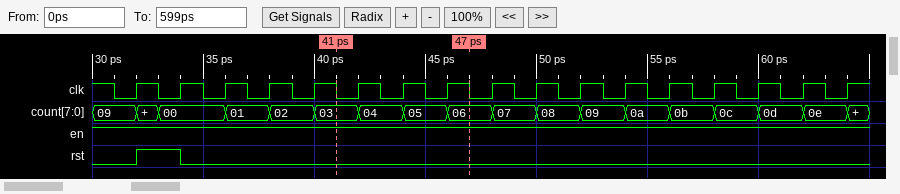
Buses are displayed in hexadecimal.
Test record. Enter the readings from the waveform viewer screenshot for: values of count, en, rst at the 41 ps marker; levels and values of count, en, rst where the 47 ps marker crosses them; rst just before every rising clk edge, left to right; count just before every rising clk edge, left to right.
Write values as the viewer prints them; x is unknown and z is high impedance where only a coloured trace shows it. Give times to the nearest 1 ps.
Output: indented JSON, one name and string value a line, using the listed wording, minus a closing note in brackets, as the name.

{
  "values of count, en, rst at the 41 ps marker": "count=03, en=1, rst=0",
  "levels and values of count, en, rst where the 47 ps marker crosses them": "count=06, en=1, rst=0",
  "rst just before every rising clk edge, left to right": "0 1 0 0 0 0 0 0 0 0 0 0 0 0 0 0 0",
  "count just before every rising clk edge, left to right": "09, 00, 00, 01, 02, 03, 04, 05, 06, 07, 08, 09, 0a, 0b, 0c, 0d, 0e"
}
